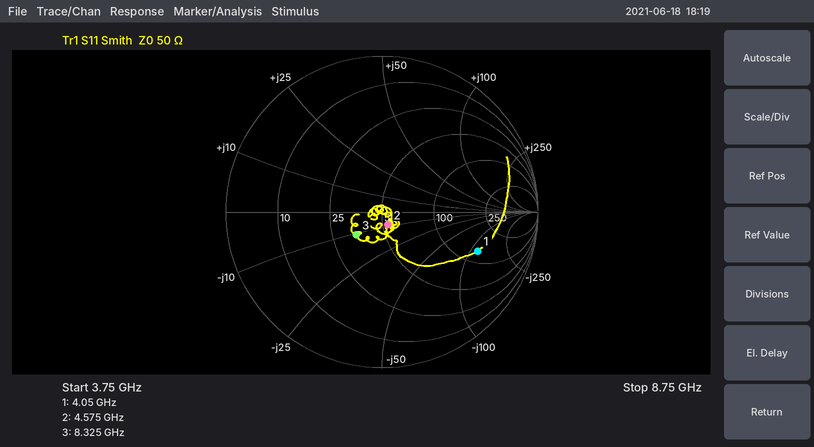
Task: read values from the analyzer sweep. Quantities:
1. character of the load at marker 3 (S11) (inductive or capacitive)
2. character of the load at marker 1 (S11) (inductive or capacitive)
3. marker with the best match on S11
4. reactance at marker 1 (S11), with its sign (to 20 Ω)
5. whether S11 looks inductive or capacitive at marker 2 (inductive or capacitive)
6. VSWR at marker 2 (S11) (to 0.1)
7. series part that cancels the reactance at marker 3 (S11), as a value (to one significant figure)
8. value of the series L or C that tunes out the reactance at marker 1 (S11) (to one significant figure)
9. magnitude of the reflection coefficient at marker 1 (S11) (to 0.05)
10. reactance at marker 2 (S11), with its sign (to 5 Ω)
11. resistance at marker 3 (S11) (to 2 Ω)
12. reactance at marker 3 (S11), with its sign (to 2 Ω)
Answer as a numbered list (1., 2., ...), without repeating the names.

1. capacitive
2. capacitive
3. marker 2
4. -120 Ω
5. capacitive
6. 1.2
7. 200 pH
8. 5 nH
9. 0.65
10. -10 Ω
11. 34 Ω
12. -10 Ω
